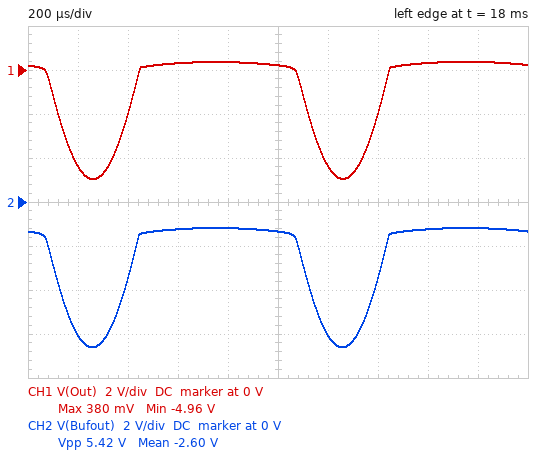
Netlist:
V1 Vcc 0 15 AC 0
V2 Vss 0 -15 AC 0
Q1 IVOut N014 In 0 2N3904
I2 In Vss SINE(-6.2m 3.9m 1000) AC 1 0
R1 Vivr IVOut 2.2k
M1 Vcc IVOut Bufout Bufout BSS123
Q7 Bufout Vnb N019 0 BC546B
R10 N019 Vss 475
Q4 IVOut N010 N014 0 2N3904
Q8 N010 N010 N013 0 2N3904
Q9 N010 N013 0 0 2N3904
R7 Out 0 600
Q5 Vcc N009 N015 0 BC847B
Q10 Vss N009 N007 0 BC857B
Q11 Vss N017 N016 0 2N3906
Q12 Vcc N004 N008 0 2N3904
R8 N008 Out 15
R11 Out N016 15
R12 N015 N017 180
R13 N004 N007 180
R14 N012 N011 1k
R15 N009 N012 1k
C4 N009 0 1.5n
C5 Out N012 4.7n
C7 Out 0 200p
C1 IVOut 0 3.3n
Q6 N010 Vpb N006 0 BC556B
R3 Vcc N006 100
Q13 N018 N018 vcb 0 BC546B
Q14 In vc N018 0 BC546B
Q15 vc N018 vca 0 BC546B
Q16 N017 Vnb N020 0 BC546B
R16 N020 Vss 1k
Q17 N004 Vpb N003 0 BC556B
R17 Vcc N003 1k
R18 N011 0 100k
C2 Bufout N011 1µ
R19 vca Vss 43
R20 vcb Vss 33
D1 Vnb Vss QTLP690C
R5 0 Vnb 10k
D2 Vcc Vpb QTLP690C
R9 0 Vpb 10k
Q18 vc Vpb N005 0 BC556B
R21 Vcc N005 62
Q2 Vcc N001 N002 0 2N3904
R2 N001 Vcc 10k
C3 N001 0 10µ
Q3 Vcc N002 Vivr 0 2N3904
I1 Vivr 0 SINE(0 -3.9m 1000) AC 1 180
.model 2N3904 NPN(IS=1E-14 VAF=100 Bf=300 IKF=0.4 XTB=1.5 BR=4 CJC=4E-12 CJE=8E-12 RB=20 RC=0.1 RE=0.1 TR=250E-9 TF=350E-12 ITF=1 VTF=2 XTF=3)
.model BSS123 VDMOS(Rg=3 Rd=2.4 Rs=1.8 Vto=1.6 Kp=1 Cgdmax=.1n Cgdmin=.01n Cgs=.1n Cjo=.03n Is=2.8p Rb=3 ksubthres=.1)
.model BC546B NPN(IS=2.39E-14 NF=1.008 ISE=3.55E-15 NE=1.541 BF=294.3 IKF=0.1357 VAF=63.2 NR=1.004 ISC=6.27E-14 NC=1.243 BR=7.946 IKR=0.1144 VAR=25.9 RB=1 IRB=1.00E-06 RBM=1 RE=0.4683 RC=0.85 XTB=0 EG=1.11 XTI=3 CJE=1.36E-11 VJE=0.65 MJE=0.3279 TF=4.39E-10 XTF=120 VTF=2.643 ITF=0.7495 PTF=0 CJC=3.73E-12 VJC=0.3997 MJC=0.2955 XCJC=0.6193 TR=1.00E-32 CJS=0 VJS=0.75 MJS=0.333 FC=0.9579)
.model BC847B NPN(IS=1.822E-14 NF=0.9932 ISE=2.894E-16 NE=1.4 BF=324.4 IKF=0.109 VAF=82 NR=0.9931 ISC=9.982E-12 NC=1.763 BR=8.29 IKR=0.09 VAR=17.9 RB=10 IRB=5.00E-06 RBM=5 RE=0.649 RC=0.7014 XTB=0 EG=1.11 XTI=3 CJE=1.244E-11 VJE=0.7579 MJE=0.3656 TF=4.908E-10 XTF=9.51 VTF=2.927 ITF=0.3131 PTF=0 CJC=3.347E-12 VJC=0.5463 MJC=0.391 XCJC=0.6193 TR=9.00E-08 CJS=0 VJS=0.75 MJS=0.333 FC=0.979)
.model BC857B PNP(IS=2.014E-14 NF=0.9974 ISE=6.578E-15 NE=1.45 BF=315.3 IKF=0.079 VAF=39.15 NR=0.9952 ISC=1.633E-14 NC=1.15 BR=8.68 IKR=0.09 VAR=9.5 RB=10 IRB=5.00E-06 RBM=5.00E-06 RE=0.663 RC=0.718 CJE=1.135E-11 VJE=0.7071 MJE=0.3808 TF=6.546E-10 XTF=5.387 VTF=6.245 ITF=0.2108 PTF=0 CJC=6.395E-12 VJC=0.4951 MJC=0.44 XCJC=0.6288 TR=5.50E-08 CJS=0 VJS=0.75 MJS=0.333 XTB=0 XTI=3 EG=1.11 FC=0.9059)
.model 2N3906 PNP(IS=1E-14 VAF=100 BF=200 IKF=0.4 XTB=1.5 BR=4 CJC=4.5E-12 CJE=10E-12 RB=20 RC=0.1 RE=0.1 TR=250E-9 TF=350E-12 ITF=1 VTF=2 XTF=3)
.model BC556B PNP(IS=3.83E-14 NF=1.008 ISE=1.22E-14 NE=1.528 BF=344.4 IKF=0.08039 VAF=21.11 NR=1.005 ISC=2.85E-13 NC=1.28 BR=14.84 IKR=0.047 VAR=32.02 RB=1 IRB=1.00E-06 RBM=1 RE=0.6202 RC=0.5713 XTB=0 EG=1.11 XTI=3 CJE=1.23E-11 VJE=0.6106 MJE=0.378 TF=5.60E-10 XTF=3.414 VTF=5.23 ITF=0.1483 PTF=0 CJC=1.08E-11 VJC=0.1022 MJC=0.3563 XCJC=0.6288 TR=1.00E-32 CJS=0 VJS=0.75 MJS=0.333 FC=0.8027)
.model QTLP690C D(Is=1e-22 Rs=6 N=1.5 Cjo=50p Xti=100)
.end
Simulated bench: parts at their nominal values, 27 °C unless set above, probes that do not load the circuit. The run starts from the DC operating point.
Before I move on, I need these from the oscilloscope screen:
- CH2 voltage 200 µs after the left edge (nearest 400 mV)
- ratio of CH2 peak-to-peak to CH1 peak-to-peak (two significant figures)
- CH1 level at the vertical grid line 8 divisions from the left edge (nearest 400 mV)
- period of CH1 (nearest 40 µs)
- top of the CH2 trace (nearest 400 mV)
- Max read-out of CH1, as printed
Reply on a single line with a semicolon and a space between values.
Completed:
-6.0 V; 1.0; 400 mV; 1.00 ms; -1.2 V; 380 mV
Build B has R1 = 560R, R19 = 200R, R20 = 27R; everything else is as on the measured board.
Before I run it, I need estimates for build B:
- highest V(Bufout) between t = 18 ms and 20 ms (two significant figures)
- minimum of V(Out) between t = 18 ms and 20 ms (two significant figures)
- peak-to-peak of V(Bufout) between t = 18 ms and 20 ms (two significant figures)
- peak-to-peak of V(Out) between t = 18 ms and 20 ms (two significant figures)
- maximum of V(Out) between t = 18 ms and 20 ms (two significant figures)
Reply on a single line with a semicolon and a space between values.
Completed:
-13 V; -100 mV; 200 mV; 190 mV; 89 mV
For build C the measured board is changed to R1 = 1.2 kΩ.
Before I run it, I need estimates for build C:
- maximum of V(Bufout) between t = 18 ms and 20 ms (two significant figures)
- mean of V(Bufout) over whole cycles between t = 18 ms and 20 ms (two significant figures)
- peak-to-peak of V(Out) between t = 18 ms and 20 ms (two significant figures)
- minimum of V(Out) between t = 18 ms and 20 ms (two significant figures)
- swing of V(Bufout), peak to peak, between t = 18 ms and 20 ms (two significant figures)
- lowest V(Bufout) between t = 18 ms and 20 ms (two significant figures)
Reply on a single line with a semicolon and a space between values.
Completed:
-970 mV; -1.1 V; 310 mV; -150 mV; 320 mV; -1.3 V
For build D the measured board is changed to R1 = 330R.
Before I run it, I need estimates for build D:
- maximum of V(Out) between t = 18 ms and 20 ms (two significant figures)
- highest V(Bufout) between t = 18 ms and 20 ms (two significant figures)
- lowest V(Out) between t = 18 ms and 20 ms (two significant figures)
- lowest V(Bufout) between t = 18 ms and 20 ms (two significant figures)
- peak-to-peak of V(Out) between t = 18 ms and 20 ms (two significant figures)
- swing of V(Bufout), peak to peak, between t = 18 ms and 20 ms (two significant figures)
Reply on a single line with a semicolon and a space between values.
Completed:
1.3 V; 8.4 V; -1.3 V; 5.9 V; 2.5 V; 2.6 V
